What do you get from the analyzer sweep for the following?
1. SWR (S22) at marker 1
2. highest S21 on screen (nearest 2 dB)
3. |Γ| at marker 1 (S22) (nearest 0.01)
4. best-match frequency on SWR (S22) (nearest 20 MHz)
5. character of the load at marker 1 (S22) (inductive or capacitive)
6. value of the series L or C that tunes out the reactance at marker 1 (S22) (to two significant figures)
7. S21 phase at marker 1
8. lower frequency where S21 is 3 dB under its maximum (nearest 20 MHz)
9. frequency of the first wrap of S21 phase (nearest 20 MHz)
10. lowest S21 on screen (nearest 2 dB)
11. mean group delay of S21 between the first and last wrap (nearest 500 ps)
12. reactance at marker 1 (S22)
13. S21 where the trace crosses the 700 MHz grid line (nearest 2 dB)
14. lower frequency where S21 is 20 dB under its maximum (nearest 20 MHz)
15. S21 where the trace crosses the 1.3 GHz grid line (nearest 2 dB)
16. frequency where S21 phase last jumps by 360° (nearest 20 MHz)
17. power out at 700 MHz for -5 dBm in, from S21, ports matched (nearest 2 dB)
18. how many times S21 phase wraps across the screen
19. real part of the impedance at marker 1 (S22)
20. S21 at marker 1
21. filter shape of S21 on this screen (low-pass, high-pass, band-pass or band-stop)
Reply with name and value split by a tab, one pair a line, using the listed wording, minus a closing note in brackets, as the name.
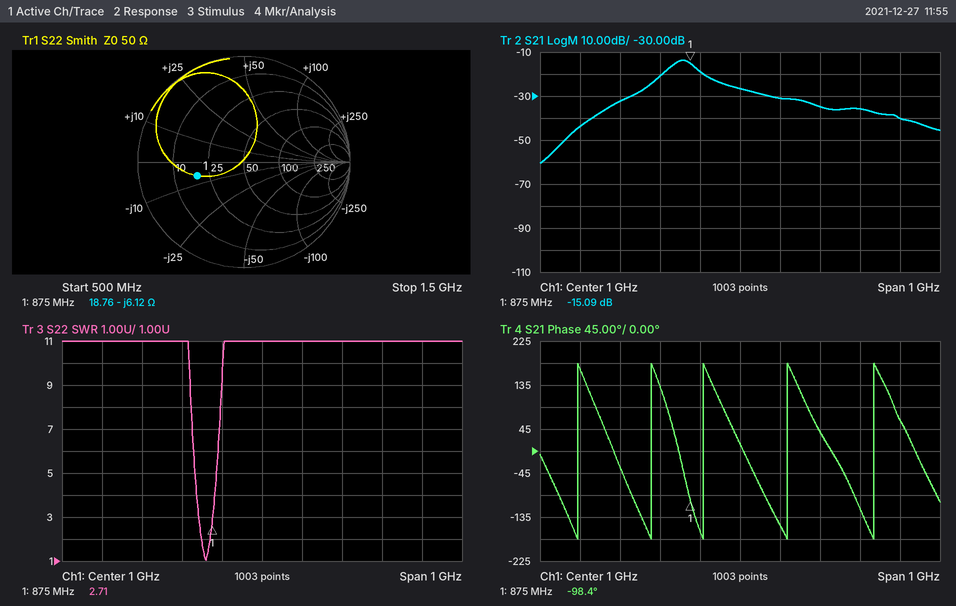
SWR (S22) at marker 1	2.71
highest S21 on screen	-14 dB
|Γ| at marker 1 (S22)	0.46
best-match frequency on SWR (S22)	860 MHz
character of the load at marker 1 (S22)	capacitive
value of the series L or C that tunes out the reactance at marker 1 (S22)	1.1 nH
S21 phase at marker 1	-98.4°
lower frequency where S21 is 3 dB under its maximum	820 MHz
frequency of the first wrap of S21 phase	600 MHz
lowest S21 on screen	-60 dB
mean group delay of S21 between the first and last wrap	5.5 ns
reactance at marker 1	-6.12 Ω
S21 where the trace crosses the 700 MHz grid line	-32 dB
lower frequency where S21 is 20 dB under its maximum	680 MHz
S21 where the trace crosses the 1.3 GHz grid line	-36 dB
frequency where S21 phase last jumps by 360°	1.34 GHz
power out at 700 MHz for -5 dBm in, from S21, ports matched	-38 dBm
how many times S21 phase wraps across the screen	5
real part of the impedance at marker 1	18.76 Ω
S21 at marker 1	-15.09 dB
filter shape of S21 on this screen	band-pass
